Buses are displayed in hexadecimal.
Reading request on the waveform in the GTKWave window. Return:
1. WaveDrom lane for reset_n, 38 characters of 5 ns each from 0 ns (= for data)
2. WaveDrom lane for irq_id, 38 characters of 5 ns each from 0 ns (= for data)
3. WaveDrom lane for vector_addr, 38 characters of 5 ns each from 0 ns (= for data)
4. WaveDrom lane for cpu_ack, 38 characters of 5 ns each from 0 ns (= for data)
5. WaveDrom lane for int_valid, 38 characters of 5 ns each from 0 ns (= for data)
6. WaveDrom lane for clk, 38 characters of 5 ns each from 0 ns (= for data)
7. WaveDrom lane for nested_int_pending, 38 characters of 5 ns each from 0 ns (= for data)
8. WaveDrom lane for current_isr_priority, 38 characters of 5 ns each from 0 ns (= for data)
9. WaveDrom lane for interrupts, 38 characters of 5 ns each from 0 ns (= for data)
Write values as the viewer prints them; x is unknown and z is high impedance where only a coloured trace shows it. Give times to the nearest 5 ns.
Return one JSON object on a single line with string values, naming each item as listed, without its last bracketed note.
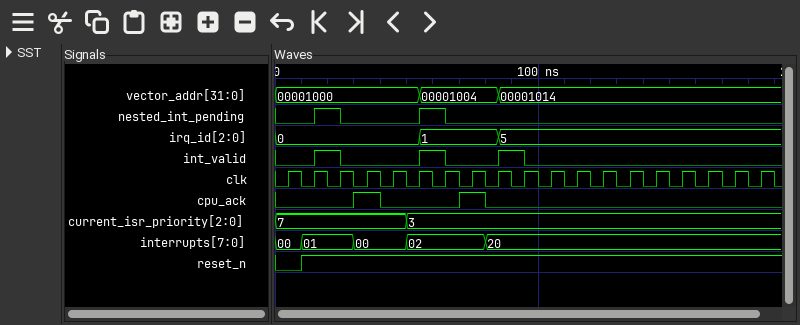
{"WaveDrom lane for reset_n, 38 characters of 5 ns each from 0 ns": "{name: 'reset_n', wave: '0.1...................................'}", "WaveDrom lane for irq_id, 38 characters of 5 ns each from 0 ns": "{name: 'irq_id', wave: '=..........=.....=....................', data: '0 1 5'}", "WaveDrom lane for vector_addr, 38 characters of 5 ns each from 0 ns": "{name: 'vector_addr', wave: '=..........=.....=....................', data: '00001000 00001004 00001014'}", "WaveDrom lane for cpu_ack, 38 characters of 5 ns each from 0 ns": "{name: 'cpu_ack', wave: '0.....1.0.....1.0.....................'}", "WaveDrom lane for int_valid, 38 characters of 5 ns each from 0 ns": "{name: 'int_valid', wave: '0..1.0.....1.0...1.0..................'}", "WaveDrom lane for clk, 38 characters of 5 ns each from 0 ns": "{name: 'clk', wave: '01010101010101010101010101010101010101'}", "WaveDrom lane for nested_int_pending, 38 characters of 5 ns each from 0 ns": "{name: 'nested_int_pending', wave: '0..1.0.....1.0........................'}", "WaveDrom lane for current_isr_priority, 38 characters of 5 ns each from 0 ns": "{name: 'current_isr_priority', wave: '=.........=...........................', data: '7 3'}", "WaveDrom lane for interrupts, 38 characters of 5 ns each from 0 ns": "{name: 'interrupts', wave: '=.=...=...=.....=.....................', data: '00 01 00 02 20'}"}
